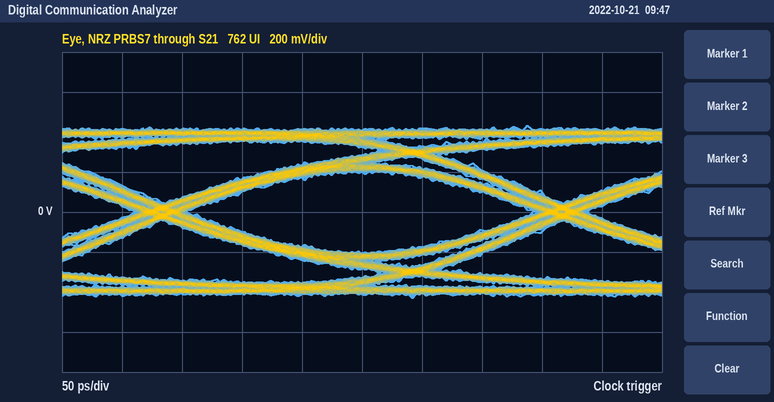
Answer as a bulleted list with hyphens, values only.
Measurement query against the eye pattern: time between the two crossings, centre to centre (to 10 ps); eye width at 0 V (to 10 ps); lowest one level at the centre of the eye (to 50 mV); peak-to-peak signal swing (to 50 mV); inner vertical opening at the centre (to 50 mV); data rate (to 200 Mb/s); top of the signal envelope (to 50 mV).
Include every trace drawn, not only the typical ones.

- 330 ps
- 290 ps
- 200 mV
- 850 mV
- 400 mV
- 3.0 Gb/s
- 450 mV
